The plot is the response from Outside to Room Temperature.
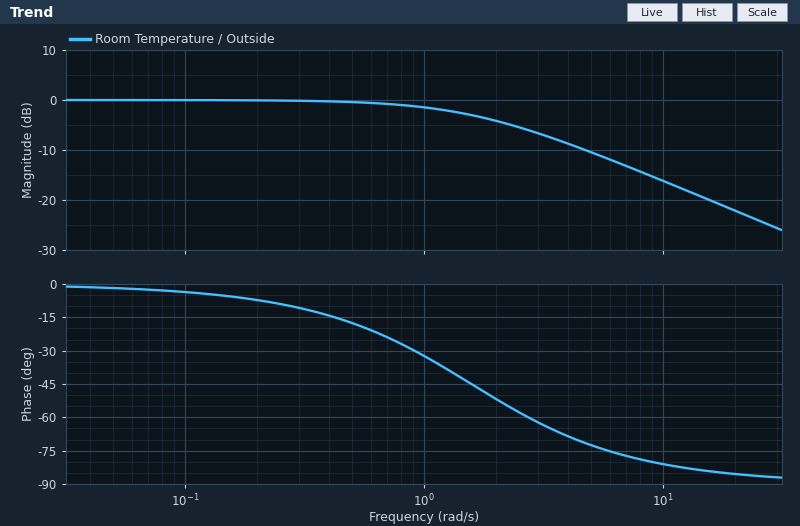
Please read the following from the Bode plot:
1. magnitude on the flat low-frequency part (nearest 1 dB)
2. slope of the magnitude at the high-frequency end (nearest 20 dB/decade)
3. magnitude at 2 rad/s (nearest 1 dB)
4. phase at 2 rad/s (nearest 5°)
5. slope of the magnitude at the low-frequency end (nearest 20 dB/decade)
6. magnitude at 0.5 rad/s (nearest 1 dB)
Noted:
0 dB
-20 dB/decade
-4 dB
-50°
0 dB/decade
0 dB
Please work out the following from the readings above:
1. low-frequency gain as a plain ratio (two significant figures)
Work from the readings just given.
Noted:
1.0
